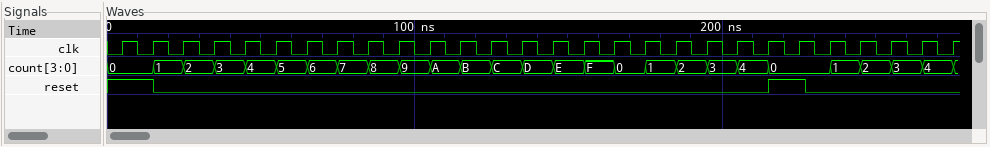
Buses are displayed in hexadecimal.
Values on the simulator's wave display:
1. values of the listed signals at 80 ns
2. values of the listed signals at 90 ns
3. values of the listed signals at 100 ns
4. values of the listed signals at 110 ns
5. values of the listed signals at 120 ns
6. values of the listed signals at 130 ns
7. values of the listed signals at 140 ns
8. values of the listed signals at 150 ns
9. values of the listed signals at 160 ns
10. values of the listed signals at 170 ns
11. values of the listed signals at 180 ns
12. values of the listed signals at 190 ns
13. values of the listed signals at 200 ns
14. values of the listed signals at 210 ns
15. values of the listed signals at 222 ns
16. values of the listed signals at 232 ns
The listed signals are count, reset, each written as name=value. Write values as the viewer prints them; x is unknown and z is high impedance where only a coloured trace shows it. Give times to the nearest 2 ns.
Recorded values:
count=7, reset=0
count=8, reset=0
count=9, reset=0
count=A, reset=0
count=B, reset=0
count=C, reset=0
count=D, reset=0
count=E, reset=0
count=F, reset=0
count=0, reset=0
count=1, reset=0
count=2, reset=0
count=3, reset=0
count=4, reset=0
count=0, reset=1
count=0, reset=0
